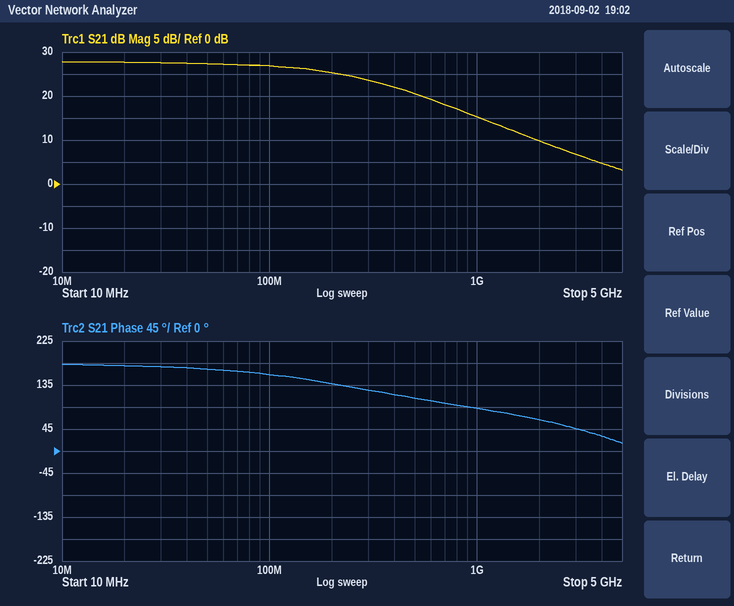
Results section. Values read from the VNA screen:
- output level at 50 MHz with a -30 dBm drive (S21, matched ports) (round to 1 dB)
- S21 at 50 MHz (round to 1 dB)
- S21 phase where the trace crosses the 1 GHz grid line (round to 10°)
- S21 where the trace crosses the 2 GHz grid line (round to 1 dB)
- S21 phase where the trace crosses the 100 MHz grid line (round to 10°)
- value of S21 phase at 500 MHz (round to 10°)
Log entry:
-3 dBm
27 dB
90°
10 dB
160°
110°
